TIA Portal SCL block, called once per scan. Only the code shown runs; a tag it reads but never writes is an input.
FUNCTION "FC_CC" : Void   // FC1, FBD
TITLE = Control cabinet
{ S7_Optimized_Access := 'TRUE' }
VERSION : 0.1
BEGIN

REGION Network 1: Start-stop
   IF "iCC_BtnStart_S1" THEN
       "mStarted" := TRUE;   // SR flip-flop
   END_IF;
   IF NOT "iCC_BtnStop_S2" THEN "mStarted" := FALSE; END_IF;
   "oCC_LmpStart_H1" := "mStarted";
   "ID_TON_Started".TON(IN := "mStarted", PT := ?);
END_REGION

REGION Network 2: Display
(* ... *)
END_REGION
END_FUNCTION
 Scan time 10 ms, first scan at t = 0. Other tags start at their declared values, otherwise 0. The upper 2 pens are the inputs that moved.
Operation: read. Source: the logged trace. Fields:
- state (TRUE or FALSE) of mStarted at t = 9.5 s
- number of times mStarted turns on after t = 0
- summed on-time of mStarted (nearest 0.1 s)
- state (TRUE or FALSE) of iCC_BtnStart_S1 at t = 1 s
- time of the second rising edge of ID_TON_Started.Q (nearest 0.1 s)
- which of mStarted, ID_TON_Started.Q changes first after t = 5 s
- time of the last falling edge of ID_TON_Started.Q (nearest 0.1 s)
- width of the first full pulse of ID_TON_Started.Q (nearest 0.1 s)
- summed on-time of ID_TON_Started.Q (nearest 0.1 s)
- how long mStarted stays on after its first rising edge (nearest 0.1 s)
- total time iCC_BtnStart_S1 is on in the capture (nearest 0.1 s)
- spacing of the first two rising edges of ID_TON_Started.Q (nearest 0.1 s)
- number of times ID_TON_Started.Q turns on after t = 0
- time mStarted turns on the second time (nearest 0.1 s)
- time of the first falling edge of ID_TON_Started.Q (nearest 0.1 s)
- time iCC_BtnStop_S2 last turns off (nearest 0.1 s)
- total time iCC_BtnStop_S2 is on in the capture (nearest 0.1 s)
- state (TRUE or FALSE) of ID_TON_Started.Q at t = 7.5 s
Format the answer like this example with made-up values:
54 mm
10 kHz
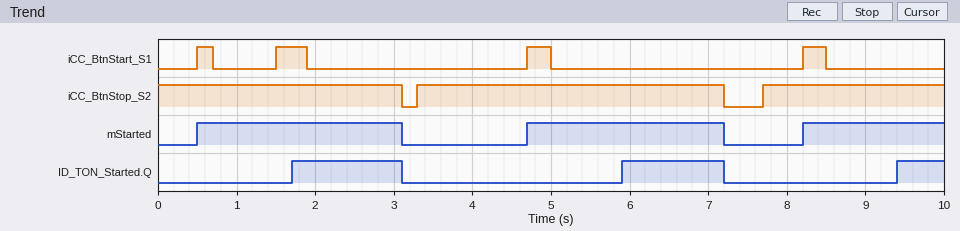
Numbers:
TRUE
3
6.9 s
FALSE
5.9 s
ID_TON_Started.Q
7.2 s
1.4 s
3.3 s
2.6 s
1.2 s
4.2 s
3
4.7 s
3.1 s
7.2 s
9.3 s
FALSE
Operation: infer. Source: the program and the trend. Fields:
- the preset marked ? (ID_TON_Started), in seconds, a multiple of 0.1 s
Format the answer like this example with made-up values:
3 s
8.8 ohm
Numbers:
1.2 s
